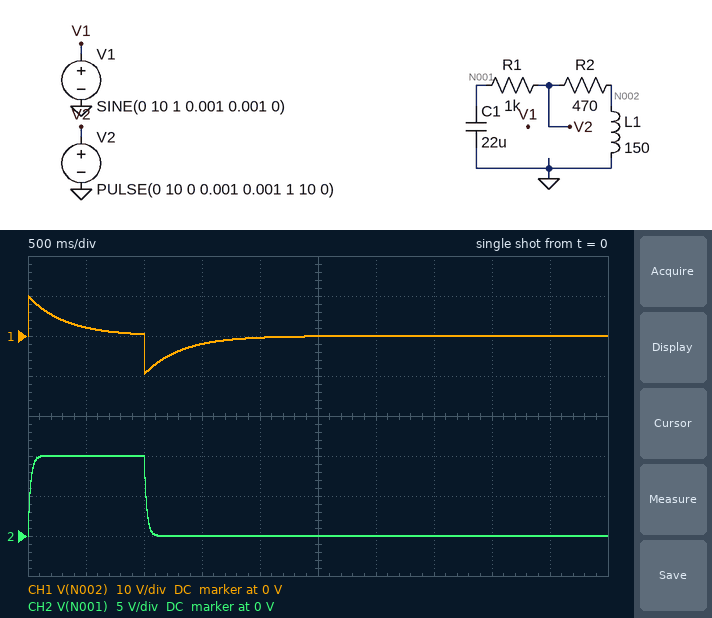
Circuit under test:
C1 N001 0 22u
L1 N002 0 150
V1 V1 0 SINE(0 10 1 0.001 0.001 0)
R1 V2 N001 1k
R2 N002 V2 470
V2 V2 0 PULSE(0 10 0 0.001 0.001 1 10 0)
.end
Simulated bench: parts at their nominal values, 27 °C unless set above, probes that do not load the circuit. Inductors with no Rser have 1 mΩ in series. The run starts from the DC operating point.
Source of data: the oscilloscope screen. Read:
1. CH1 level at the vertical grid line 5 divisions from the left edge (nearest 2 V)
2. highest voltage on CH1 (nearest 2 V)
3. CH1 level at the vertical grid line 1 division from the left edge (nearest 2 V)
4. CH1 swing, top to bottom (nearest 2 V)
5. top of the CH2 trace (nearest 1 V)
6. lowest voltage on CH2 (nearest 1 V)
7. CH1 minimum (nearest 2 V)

0 V
10 V
2 V
20 V
10 V
0 V
-10 V
